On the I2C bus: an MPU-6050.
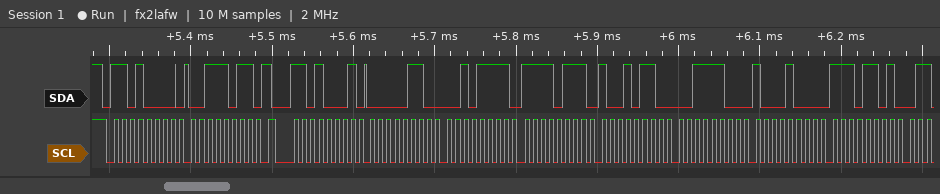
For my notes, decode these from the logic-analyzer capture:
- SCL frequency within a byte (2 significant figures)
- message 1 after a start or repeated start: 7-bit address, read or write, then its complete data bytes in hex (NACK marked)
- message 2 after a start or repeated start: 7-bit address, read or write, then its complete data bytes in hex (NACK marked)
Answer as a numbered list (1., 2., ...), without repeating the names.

1. 100 kHz
2. 0x68 write: 3B
3. 0x68 read: 06 2F F7 96 3C 88 ED
